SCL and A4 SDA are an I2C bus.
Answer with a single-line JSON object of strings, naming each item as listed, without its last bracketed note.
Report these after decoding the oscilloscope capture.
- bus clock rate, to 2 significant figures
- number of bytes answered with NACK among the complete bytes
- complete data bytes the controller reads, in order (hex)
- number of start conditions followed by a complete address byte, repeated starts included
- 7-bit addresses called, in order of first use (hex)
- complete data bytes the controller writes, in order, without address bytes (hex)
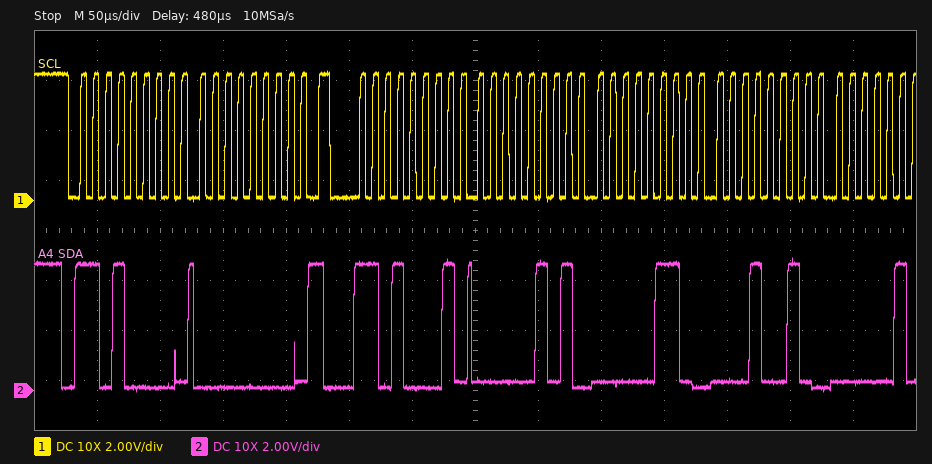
{"bus clock rate, to 2 significant figures": "100 kHz", "number of bytes answered with NACK among the complete bytes": "0", "complete data bytes the controller reads, in order": "05 06 12", "number of start conditions followed by a complete address byte, repeated starts included": "2", "7-bit addresses called, in order of first use": "0x68", "complete data bytes the controller writes, in order, without address bytes": "00"}
